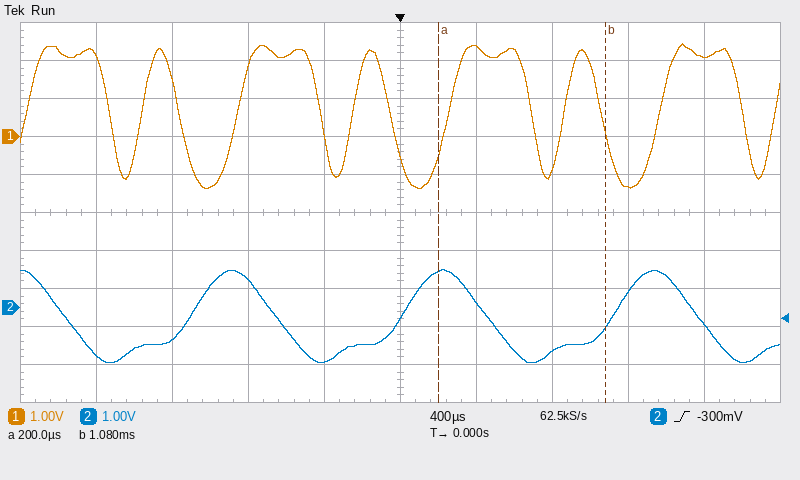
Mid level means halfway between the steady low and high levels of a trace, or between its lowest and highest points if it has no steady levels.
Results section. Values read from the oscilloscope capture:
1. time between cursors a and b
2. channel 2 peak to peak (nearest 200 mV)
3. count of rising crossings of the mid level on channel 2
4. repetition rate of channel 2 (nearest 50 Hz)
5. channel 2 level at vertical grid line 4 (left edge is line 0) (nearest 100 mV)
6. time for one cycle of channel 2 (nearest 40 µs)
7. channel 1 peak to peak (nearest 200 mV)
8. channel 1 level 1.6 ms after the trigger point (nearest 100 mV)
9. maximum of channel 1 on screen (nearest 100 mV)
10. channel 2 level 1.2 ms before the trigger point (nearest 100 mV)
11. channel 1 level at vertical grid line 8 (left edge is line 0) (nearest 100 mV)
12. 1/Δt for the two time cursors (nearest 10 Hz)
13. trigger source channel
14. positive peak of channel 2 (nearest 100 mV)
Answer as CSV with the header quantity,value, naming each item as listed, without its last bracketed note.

quantity,value
time between cursors a and b,880 µs
channel 2 peak to peak,2.4 V
count of rising crossings of the mid level on channel 2,3
repetition rate of channel 2,900 Hz
channel 2 level at vertical grid line 4 (left edge is line 0),-1.4 V
time for one cycle of channel 2,1.12 ms
channel 1 peak to peak,3.8 V
channel 1 level 1.6 ms after the trigger point,2.1 V
maximum of channel 1 on screen,2.4 V
channel 2 level 1.2 ms before the trigger point,-800 mV
channel 1 level at vertical grid line 8 (left edge is line 0),-1.3 V
1/Δt for the two time cursors,1.14 kHz
trigger source channel,channel 2
positive peak of channel 2,1.0 V
